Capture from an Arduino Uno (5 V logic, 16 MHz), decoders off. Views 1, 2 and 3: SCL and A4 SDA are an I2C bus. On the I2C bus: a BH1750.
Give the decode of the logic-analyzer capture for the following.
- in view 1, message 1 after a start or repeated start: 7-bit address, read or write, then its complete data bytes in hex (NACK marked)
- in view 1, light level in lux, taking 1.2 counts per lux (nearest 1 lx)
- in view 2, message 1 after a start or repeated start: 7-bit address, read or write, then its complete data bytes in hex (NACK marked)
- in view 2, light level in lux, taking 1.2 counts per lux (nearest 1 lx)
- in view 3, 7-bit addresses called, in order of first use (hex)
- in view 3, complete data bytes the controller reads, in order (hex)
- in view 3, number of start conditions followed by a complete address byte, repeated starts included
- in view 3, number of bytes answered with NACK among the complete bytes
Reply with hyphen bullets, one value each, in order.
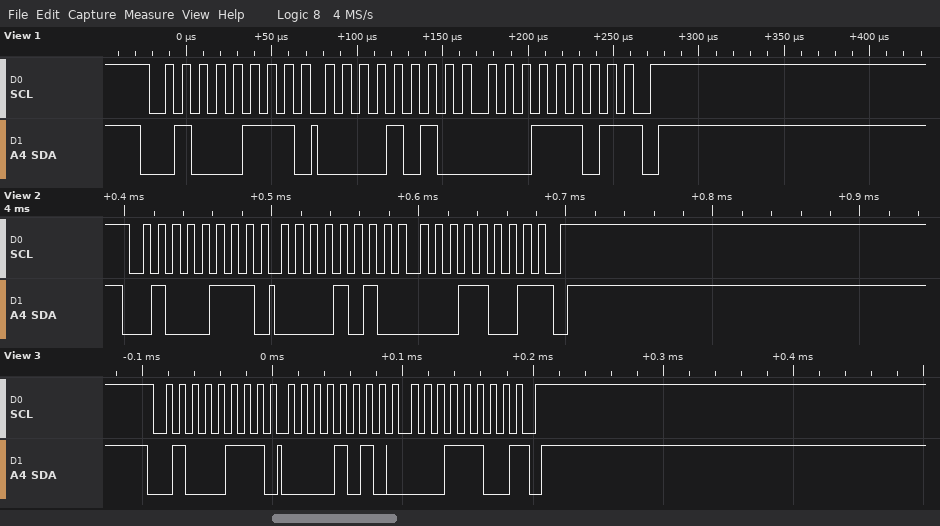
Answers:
- 0x23 read: 0A 1D NACK
- 2158 lx
- 0x23 read: 0A 19 NACK
- 2154 lx
- 0x23
- 0A 1C
- 1
- 1
